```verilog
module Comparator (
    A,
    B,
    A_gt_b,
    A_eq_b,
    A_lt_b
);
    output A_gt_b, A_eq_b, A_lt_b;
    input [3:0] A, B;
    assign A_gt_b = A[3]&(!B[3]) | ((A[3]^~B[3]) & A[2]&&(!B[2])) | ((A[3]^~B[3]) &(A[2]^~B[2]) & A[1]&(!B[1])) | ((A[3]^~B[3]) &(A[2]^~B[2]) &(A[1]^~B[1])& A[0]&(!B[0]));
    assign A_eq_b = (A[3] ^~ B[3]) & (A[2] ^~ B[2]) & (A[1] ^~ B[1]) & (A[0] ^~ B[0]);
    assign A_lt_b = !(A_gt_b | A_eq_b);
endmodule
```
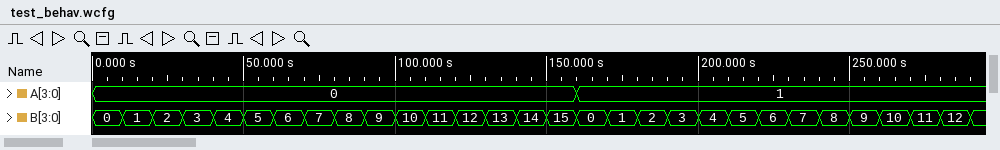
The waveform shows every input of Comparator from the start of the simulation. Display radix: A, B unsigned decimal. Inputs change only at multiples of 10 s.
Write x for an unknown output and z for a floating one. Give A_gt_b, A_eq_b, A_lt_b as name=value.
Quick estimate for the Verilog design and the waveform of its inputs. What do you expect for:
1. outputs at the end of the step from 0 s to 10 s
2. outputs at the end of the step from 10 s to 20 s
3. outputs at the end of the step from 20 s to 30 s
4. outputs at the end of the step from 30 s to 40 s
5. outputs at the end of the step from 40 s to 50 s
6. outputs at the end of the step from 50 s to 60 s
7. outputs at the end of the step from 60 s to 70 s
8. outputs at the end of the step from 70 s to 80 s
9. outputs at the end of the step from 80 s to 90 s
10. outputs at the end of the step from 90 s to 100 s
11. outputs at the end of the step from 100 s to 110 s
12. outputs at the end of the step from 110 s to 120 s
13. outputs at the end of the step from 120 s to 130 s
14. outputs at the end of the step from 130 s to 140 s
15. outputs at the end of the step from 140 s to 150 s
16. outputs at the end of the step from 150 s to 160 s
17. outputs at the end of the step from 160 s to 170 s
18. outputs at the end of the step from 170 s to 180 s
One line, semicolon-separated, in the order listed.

A_gt_b=0, A_eq_b=1, A_lt_b=0; A_gt_b=0, A_eq_b=0, A_lt_b=1; A_gt_b=0, A_eq_b=0, A_lt_b=1; A_gt_b=0, A_eq_b=0, A_lt_b=1; A_gt_b=0, A_eq_b=0, A_lt_b=1; A_gt_b=0, A_eq_b=0, A_lt_b=1; A_gt_b=0, A_eq_b=0, A_lt_b=1; A_gt_b=0, A_eq_b=0, A_lt_b=1; A_gt_b=0, A_eq_b=0, A_lt_b=1; A_gt_b=0, A_eq_b=0, A_lt_b=1; A_gt_b=0, A_eq_b=0, A_lt_b=1; A_gt_b=0, A_eq_b=0, A_lt_b=1; A_gt_b=0, A_eq_b=0, A_lt_b=1; A_gt_b=0, A_eq_b=0, A_lt_b=1; A_gt_b=0, A_eq_b=0, A_lt_b=1; A_gt_b=0, A_eq_b=0, A_lt_b=1; A_gt_b=1, A_eq_b=0, A_lt_b=0; A_gt_b=0, A_eq_b=1, A_lt_b=0
